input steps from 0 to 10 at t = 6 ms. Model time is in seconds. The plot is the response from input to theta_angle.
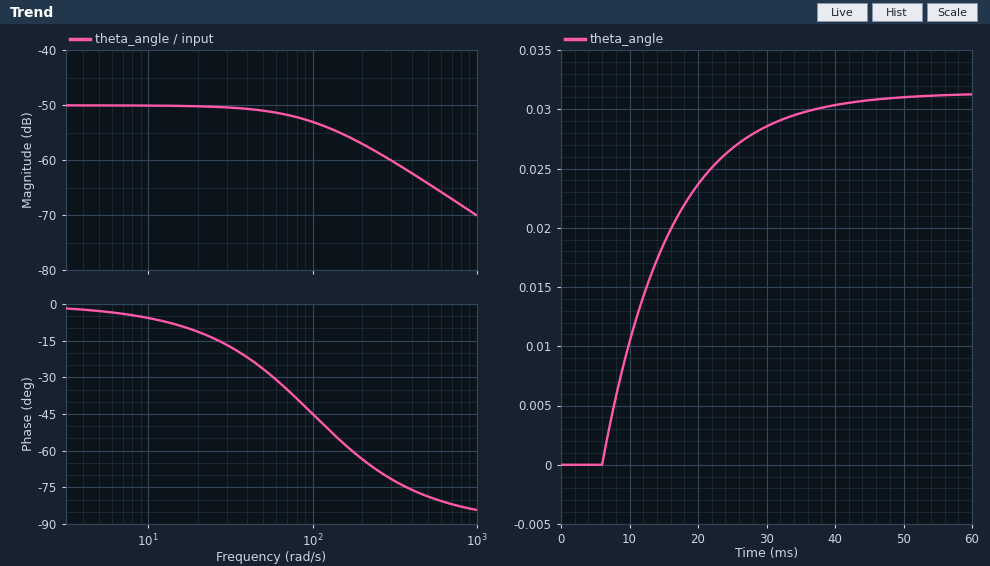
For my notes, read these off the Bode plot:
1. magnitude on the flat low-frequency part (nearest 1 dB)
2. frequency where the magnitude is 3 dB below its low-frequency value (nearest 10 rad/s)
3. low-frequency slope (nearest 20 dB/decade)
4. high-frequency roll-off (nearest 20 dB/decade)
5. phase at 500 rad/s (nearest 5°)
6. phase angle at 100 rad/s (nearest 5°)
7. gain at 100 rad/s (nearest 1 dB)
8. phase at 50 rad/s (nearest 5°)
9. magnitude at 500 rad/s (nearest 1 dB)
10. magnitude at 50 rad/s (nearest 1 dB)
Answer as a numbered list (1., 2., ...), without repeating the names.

1. -50 dB
2. 100 rad/s
3. 0 dB/decade
4. -20 dB/decade
5. -80°
6. -45°
7. -53 dB
8. -25°
9. -64 dB
10. -51 dB
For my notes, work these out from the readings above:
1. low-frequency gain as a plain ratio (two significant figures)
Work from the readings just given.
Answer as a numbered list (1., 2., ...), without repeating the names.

1. 0.0032
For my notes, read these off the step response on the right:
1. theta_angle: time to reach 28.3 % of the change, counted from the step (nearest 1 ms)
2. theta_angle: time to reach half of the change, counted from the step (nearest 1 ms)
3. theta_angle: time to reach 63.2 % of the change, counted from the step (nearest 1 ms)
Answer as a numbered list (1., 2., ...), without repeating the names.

1. 3 ms
2. 7 ms
3. 10 ms
